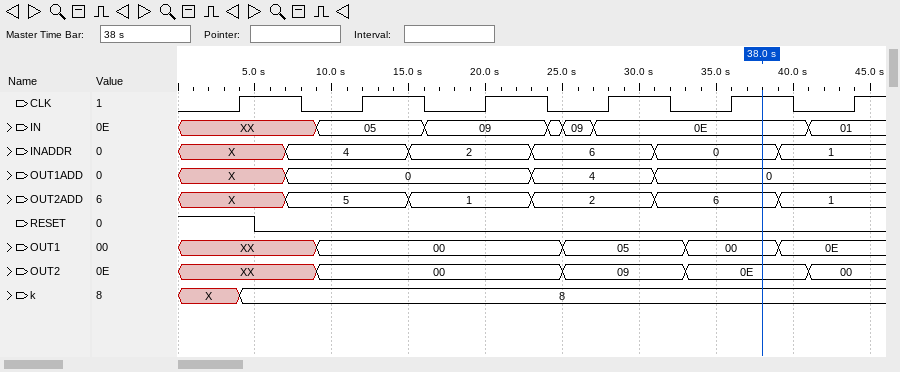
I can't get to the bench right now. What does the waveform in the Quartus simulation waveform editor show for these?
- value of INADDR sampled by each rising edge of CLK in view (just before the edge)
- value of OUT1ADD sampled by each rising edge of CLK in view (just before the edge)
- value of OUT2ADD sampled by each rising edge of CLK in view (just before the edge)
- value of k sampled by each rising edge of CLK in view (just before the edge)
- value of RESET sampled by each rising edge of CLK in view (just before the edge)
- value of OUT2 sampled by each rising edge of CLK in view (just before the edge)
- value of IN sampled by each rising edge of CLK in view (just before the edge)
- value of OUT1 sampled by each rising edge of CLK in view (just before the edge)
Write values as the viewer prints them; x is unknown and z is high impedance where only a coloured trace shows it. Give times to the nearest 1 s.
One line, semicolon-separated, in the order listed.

X, 4, 2, 6, 0, 1; X, 0, 0, 4, 0, 0; X, 5, 1, 2, 6, 1; X, 8, 8, 8, 8, 8; 1 0 0 0 0 0; XX, 00, 00, 09, 0E, 00; XX, 05, 09, 0E, 0E, 01; XX, 00, 00, 05, 00, 0E
